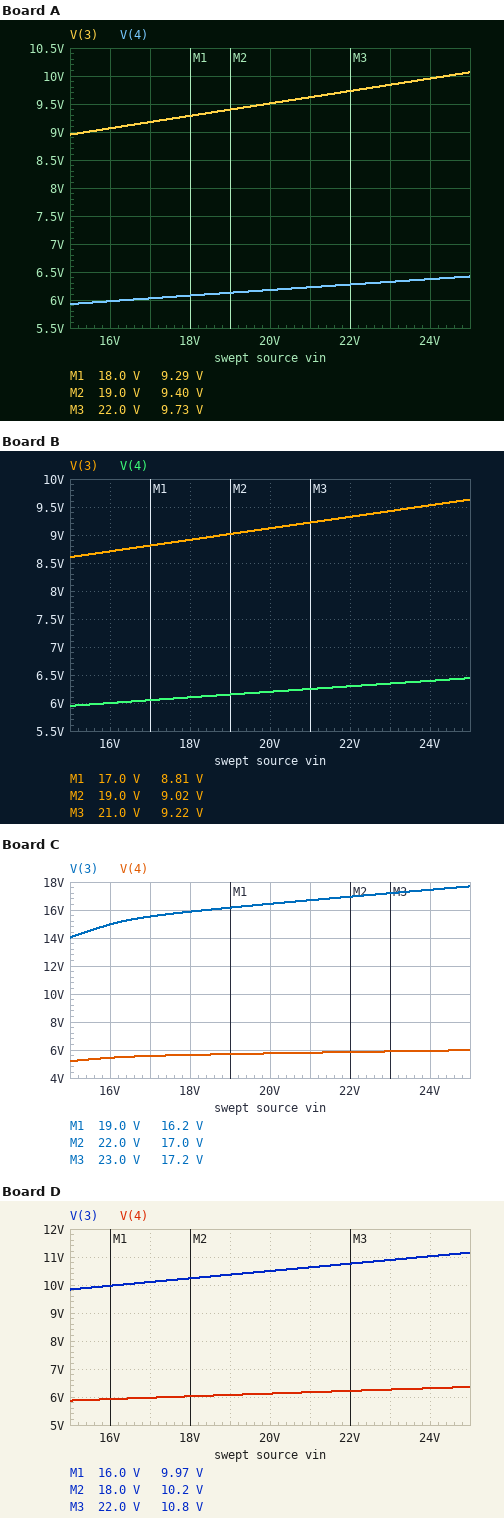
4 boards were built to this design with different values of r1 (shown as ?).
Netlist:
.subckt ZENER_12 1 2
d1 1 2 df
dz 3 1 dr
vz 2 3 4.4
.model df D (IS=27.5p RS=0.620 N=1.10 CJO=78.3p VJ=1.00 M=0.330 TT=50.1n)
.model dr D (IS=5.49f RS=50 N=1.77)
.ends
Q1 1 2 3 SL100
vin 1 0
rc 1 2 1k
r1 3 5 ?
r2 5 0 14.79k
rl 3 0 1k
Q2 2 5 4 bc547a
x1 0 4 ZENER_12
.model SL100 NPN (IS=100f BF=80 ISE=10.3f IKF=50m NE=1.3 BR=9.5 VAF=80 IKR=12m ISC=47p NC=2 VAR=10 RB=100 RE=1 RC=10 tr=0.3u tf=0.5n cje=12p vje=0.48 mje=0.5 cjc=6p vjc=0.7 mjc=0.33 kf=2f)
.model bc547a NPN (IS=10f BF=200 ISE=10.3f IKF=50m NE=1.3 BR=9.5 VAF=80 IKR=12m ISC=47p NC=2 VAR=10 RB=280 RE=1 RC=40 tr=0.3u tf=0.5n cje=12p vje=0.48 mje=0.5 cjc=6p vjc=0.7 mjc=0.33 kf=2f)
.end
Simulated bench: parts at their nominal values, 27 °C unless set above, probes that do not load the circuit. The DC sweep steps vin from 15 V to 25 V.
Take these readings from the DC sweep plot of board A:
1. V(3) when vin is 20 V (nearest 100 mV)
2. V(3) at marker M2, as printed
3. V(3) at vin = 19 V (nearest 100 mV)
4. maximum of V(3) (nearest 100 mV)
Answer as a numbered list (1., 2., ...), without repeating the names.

1. 9.5 V
2. 9.40 V
3. 9.4 V
4. 10.1 V
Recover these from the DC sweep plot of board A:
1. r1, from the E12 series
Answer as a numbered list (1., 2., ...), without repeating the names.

1. 4.7 kΩ
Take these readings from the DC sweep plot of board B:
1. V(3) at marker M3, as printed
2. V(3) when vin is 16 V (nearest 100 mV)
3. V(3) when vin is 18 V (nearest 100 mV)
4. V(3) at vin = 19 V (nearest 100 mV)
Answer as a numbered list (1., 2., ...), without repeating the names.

1. 9.22 V
2. 8.7 V
3. 8.9 V
4. 9.0 V
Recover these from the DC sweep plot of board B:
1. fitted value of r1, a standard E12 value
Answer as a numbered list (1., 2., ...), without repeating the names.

1. 3.9 kΩ
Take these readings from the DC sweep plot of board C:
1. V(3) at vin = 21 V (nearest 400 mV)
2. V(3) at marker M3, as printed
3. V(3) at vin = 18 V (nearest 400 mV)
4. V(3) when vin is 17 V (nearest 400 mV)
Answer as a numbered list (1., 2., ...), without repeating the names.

1. 16.8 V
2. 17.2 V
3. 16.0 V
4. 15.6 V
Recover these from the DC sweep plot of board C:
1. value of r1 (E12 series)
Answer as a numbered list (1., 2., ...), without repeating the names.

1. 22 kΩ
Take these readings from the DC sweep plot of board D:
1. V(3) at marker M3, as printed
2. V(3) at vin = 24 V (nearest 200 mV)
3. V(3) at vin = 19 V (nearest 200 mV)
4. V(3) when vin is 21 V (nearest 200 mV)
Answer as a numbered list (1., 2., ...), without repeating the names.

1. 10.8 V
2. 11.0 V
3. 10.4 V
4. 10.6 V
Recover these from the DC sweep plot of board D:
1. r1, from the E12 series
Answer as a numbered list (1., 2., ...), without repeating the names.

1. 6.8 kΩ
